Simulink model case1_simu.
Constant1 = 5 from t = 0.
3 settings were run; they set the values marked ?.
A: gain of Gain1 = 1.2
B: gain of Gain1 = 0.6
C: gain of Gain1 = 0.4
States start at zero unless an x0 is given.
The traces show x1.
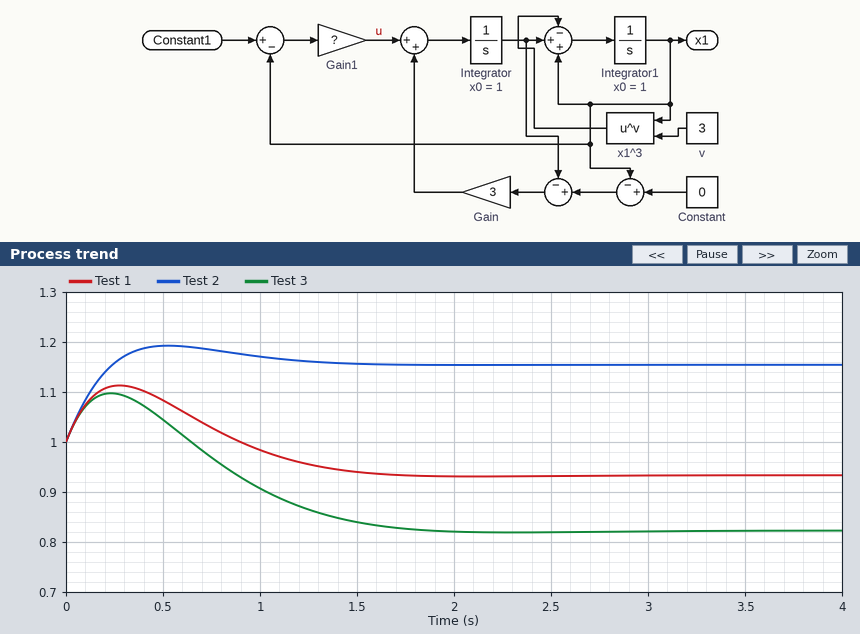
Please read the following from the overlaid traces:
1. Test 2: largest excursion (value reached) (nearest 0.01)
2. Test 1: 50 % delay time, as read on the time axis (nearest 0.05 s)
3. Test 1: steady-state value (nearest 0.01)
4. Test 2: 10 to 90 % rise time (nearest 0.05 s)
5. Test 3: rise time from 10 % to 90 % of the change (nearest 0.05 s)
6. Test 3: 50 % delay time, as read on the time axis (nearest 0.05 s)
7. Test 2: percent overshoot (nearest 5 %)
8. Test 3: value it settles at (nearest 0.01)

1.19
1.15 s
0.93
0.20 s
0.80 s
1.00 s
25 %
0.82
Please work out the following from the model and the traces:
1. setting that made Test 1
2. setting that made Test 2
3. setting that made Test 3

B
A
C
